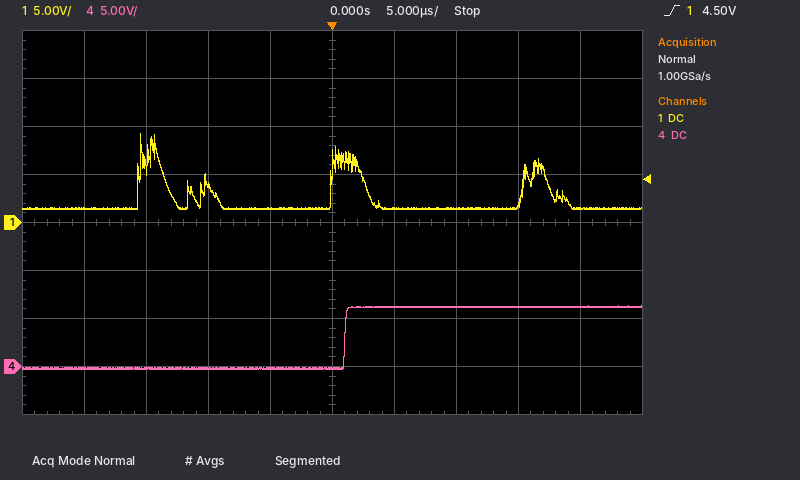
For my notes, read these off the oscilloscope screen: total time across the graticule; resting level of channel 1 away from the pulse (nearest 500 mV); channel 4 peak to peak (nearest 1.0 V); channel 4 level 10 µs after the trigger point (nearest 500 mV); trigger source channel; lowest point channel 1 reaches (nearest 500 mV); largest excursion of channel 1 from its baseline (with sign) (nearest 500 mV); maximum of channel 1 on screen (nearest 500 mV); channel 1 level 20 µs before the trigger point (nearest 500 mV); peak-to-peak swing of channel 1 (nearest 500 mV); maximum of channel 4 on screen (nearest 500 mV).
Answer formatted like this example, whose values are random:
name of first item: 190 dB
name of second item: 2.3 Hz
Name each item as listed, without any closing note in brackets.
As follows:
total time across the graticule: 50 µs
resting level of channel 1 away from the pulse: 1.5 V
channel 4 peak to peak: 7.0 V
channel 4 level 10 µs after the trigger point: 6.0 V
trigger source channel: channel 1
lowest point channel 1 reaches: 1.5 V
largest excursion of channel 1 from its baseline (with sign): +8.0 V
maximum of channel 1 on screen: 9.5 V
channel 1 level 20 µs before the trigger point: 1.5 V
peak-to-peak swing of channel 1: 8.0 V
maximum of channel 4 on screen: 6.5 V
